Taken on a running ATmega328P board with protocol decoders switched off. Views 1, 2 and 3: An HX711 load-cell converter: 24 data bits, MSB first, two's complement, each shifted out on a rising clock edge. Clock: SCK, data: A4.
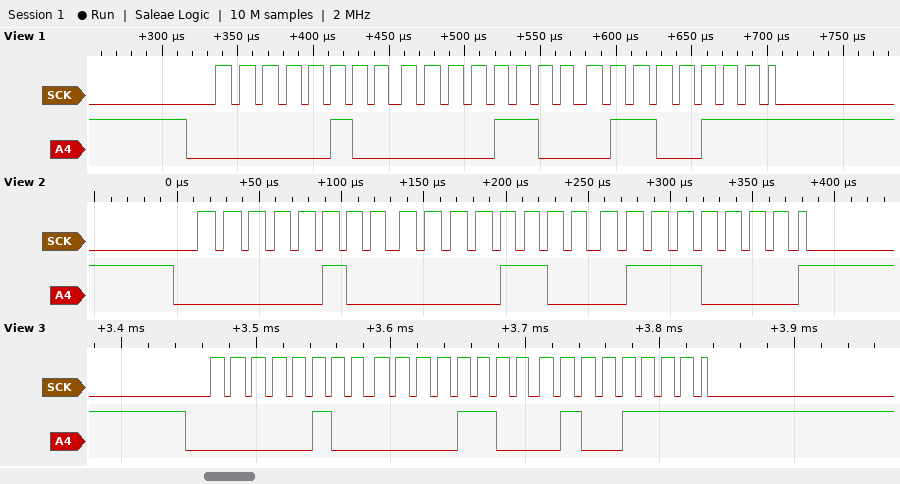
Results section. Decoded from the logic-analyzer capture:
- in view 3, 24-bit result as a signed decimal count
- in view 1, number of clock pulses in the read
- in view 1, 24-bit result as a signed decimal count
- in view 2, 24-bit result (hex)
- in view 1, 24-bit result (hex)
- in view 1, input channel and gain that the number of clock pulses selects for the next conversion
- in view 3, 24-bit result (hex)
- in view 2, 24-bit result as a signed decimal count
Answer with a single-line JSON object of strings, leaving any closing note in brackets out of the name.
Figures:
{"in view 3, 24-bit result as a signed decimal count": "265295", "in view 1, number of clock pulses in the read": "25", "in view 1, 24-bit result as a signed decimal count": "265319", "in view 2, 24-bit result": "0x040C70", "in view 1, 24-bit result": "0x040C67", "in view 1, input channel and gain that the number of clock pulses selects for the next conversion": "channel A, gain 128", "in view 3, 24-bit result": "0x040C4F", "in view 2, 24-bit result as a signed decimal count": "265328"}
